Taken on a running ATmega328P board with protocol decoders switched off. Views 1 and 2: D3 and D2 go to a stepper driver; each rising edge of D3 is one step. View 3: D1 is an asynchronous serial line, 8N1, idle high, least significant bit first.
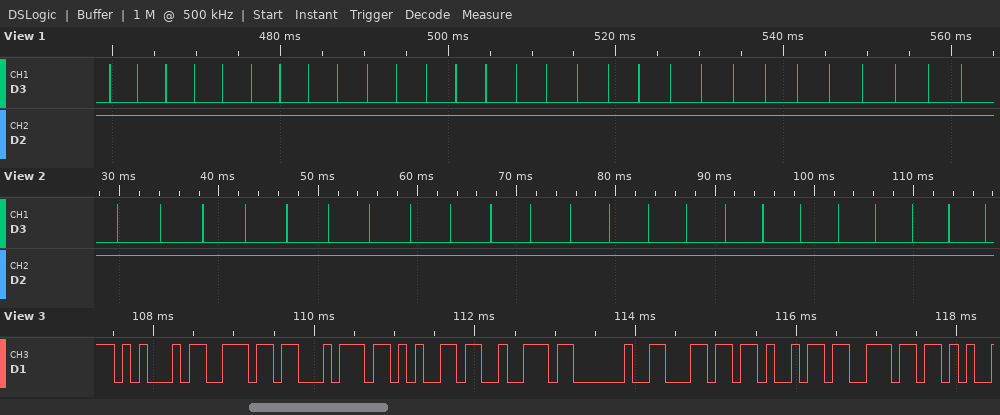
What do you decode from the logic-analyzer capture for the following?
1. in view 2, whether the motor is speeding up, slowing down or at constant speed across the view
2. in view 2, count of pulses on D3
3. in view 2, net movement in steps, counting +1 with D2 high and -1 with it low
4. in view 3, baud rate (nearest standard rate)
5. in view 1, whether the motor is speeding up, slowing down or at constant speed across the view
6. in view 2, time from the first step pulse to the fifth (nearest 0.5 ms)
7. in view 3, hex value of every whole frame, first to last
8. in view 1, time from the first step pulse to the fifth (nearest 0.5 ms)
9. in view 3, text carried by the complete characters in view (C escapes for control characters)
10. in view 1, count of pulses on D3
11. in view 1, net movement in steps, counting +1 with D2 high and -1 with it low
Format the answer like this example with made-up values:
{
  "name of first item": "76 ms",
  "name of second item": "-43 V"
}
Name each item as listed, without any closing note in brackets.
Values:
{
  "in view 2, whether the motor is speeding up, slowing down or at constant speed across the view": "speeding up",
  "in view 2, count of pulses on D3": "23",
  "in view 2, net movement in steps, counting +1 with D2 high and -1 with it low": "+23",
  "in view 3, baud rate": "9600 baud",
  "in view 1, whether the motor is speeding up, slowing down or at constant speed across the view": "slowing down",
  "in view 2, time from the first step pulse to the fifth": "17.0 ms",
  "in view 3, hex value of every whole frame, first to last": "45 6E 74 65 72 20 6C 69 6E",
  "in view 1, time from the first step pulse to the fifth": "13.5 ms",
  "in view 3, text carried by the complete characters in view": "\"Enter lin\"",
  "in view 1, count of pulses on D3": "29",
  "in view 1, net movement in steps, counting +1 with D2 high and -1 with it low": "+29"
}
